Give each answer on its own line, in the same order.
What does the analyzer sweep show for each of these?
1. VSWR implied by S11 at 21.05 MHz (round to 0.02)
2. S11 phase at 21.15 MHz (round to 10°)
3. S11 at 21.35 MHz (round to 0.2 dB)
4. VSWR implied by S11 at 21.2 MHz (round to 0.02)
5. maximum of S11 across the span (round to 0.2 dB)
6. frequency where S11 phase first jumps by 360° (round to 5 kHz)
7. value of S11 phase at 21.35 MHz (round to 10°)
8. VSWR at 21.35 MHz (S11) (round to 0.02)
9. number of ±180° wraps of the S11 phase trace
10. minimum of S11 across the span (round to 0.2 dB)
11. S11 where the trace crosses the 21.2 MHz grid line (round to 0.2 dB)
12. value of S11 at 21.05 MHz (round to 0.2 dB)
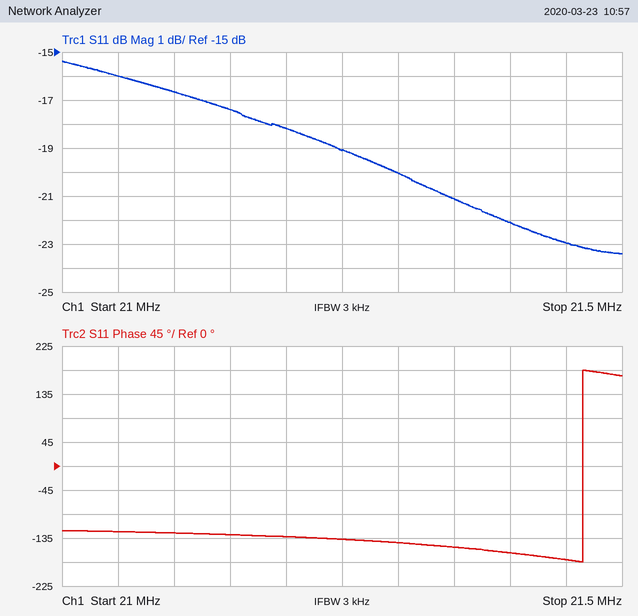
1.38
-130°
-21.2 dB
1.28
-15.4 dB
21.465 MHz
-150°
1.20
1
-23.4 dB
-18.2 dB
-16.0 dB
